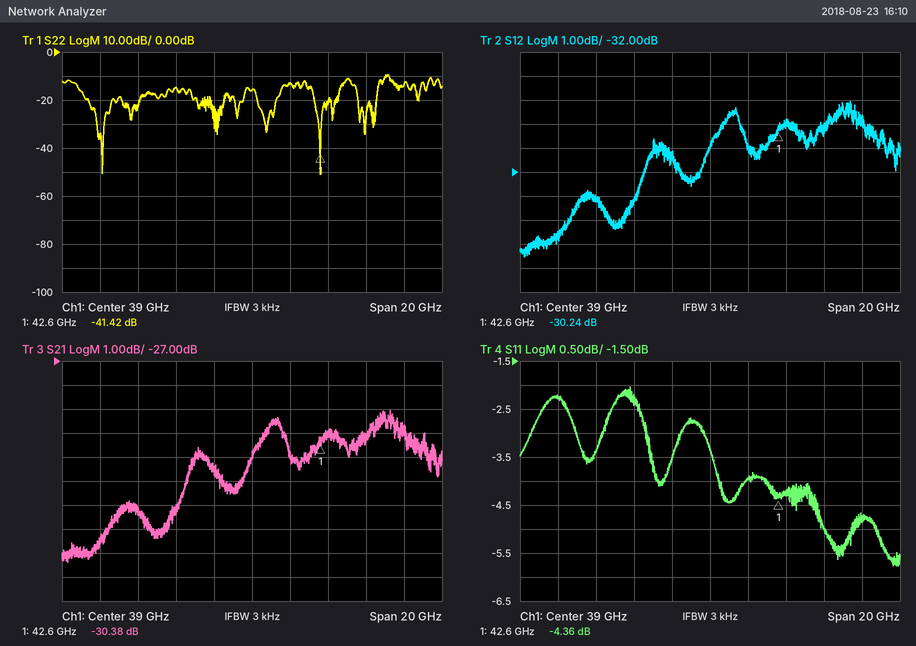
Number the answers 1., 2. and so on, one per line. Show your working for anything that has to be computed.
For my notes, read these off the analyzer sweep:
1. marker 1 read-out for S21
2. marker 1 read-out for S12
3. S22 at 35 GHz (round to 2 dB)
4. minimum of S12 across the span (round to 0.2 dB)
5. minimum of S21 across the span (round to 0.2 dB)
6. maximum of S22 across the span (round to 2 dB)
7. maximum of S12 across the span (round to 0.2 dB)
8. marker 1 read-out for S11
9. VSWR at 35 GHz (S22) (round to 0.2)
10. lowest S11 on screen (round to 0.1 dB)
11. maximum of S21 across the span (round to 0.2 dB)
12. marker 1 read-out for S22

1. -30.38 dB
2. -30.24 dB
3. -14 dB
4. -35.6 dB
5. -35.4 dB
6. -10 dB
7. -29.0 dB
8. -4.36 dB
9. |Γ| = 10^(-14/20) = 0.1995; VSWR = (1 + 0.1995)/(1 − 0.1995) ≈ 1.50, so 1.4 to the nearest 0.2
10. -5.8 dB
11. -29.0 dB
12. -41.42 dB
